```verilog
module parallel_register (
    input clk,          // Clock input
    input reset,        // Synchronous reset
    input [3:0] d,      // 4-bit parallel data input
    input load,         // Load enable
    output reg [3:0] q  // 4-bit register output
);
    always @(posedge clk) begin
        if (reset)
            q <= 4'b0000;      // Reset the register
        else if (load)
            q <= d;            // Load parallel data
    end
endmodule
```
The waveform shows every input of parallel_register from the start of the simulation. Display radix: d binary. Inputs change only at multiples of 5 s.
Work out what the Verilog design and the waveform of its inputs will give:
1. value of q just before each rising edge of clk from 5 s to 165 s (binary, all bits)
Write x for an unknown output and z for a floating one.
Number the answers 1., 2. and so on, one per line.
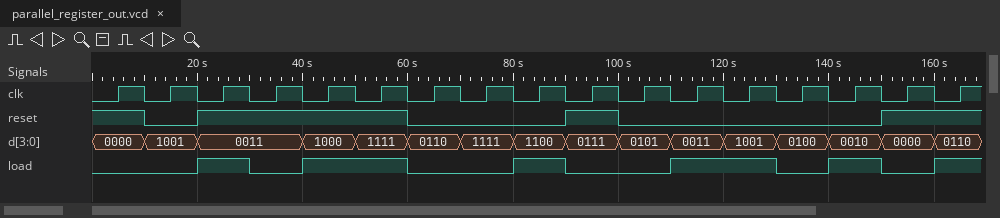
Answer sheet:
1. x, 0000, 0000, 0000, 0000, 0000, 0000, 0000, 0000, 1100, 0000, 0000, 0011, 1001, 1001, 0010, 0000
